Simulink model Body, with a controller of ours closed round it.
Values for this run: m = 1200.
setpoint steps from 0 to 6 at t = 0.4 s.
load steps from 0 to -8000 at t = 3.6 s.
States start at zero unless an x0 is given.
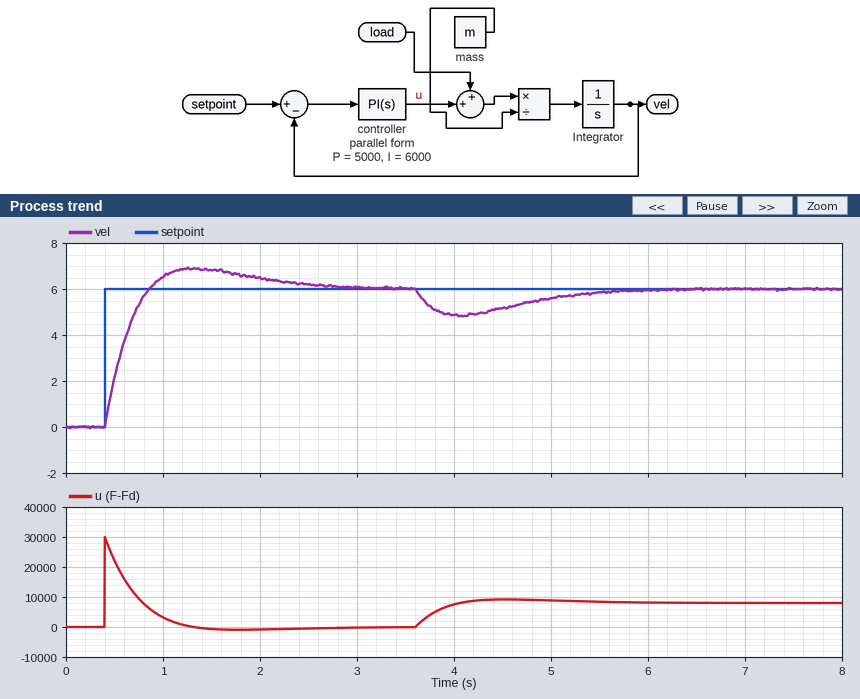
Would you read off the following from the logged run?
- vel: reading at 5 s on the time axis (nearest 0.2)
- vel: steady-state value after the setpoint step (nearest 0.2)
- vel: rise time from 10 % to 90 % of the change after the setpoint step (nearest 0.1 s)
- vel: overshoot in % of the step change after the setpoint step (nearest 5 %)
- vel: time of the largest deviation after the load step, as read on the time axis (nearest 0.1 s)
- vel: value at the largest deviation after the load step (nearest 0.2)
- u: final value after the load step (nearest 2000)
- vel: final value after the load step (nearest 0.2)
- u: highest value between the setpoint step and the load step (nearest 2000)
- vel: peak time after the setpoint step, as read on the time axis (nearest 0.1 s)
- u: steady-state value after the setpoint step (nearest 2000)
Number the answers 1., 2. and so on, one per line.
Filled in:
1. 5.6
2. 6.0
3. 0.3 s
4. 15 %
5. 4.1 s
6. 4.8
7. 8000
8. 6.0
9. 30000
10. 1.3 s
11. 0
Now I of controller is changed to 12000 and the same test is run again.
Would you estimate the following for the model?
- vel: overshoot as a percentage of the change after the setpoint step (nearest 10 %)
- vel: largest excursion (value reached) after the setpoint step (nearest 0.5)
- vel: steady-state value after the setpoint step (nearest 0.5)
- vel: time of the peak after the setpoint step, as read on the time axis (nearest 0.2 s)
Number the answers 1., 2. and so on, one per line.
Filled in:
1. 20 %
2. 7.5
3. 6.0
4. 1.2 s
